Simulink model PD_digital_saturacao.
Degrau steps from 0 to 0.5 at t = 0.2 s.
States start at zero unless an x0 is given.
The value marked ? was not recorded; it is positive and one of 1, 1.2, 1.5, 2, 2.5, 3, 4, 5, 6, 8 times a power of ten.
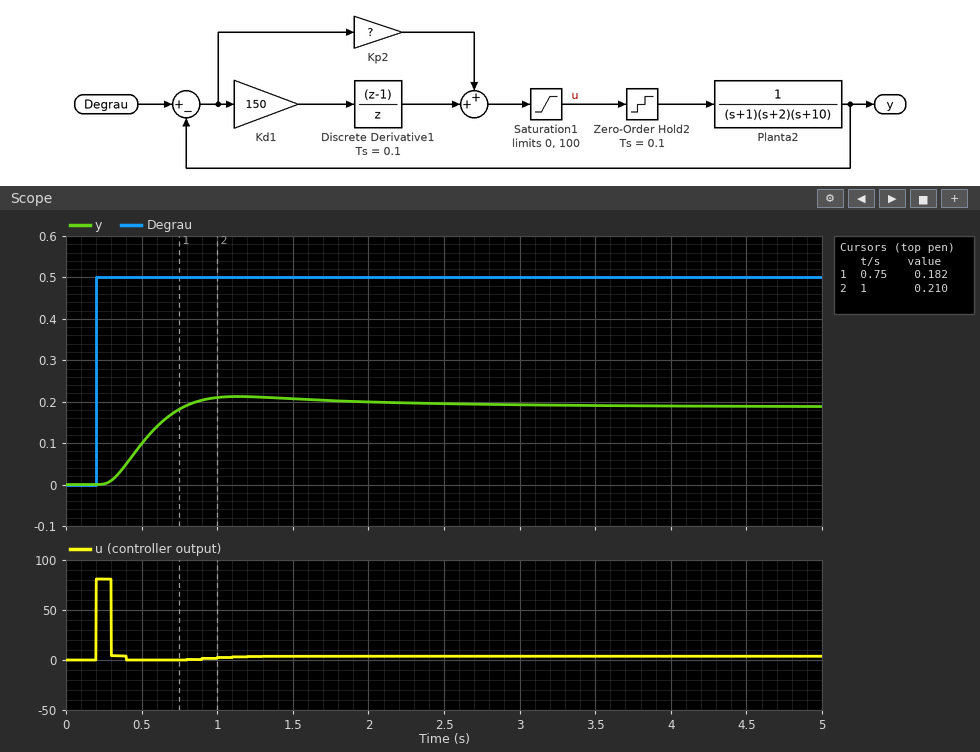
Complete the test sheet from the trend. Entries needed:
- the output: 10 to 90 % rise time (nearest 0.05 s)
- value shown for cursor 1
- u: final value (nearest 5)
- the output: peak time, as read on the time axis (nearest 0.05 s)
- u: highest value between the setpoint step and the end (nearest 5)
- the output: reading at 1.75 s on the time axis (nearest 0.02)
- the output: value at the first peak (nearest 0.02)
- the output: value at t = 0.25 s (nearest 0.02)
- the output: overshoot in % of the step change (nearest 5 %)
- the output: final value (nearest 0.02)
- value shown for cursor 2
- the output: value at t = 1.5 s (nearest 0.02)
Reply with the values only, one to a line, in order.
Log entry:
0.35 s
0.182
5
1.15 s
80
0.20
0.22
0.00
15 %
0.18
0.210
0.20
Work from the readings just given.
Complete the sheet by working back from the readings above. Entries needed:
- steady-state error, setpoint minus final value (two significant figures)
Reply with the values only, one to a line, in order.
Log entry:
0.32
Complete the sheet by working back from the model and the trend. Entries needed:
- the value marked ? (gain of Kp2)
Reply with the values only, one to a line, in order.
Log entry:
12
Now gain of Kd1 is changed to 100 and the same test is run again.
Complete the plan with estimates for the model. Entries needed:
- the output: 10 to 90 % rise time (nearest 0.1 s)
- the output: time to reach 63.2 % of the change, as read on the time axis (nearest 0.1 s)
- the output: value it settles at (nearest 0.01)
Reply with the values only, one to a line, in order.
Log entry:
0.7 s
0.7 s
0.19
